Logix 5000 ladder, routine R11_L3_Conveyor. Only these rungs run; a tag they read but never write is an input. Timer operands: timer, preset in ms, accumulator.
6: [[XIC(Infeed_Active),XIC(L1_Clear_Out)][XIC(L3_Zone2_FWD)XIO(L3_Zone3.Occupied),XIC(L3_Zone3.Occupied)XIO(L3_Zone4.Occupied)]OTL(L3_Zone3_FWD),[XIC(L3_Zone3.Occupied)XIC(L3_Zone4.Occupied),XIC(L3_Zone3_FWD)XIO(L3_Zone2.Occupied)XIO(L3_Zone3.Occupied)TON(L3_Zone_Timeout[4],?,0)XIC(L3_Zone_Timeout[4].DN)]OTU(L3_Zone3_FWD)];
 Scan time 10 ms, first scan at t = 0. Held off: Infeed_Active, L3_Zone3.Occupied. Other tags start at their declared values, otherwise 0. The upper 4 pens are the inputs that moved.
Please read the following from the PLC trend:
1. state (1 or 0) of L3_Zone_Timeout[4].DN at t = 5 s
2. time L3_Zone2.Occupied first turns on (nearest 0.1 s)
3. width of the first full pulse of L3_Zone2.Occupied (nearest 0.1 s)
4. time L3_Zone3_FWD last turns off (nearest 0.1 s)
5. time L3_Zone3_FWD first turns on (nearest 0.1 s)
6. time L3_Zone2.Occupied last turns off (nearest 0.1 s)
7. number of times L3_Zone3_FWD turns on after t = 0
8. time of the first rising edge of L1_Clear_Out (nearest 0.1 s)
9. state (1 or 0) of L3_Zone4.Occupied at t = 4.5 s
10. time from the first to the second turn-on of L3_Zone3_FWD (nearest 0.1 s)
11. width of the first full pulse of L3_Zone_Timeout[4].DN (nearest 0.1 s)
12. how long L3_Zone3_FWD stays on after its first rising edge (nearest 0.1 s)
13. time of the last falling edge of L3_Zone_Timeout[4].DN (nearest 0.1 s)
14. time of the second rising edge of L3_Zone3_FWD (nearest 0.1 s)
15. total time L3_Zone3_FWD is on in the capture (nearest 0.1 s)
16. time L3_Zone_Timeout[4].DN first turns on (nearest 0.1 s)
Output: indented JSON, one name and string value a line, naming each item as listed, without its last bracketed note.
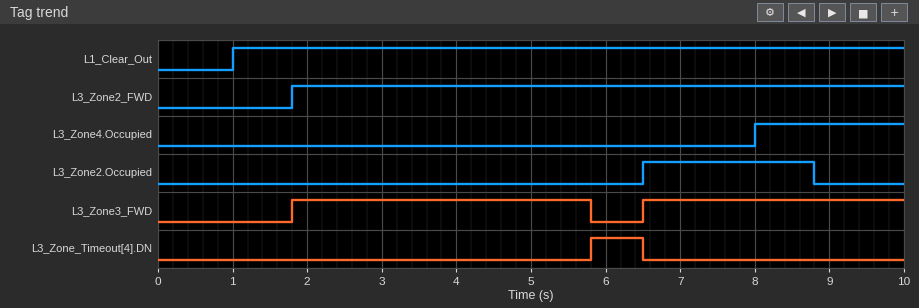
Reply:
{
  "state (1 or 0) of L3_Zone_Timeout[4].DN at t = 5 s": "0",
  "time L3_Zone2.Occupied first turns on": "6.5 s",
  "width of the first full pulse of L3_Zone2.Occupied": "2.3 s",
  "time L3_Zone3_FWD last turns off": "5.8 s",
  "time L3_Zone3_FWD first turns on": "1.8 s",
  "time L3_Zone2.Occupied last turns off": "8.8 s",
  "number of times L3_Zone3_FWD turns on after t = 0": "2",
  "time of the first rising edge of L1_Clear_Out": "1.0 s",
  "state (1 or 0) of L3_Zone4.Occupied at t = 4.5 s": "0",
  "time from the first to the second turn-on of L3_Zone3_FWD": "4.7 s",
  "width of the first full pulse of L3_Zone_Timeout[4].DN": "0.7 s",
  "how long L3_Zone3_FWD stays on after its first rising edge": "4.0 s",
  "time of the last falling edge of L3_Zone_Timeout[4].DN": "6.5 s",
  "time of the second rising edge of L3_Zone3_FWD": "6.5 s",
  "total time L3_Zone3_FWD is on in the capture": "7.5 s",
  "time L3_Zone_Timeout[4].DN first turns on": "5.8 s"
}
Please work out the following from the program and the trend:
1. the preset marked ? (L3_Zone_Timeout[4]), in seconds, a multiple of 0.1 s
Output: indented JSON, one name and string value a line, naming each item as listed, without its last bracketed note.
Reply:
{
  "the preset marked ? (L3_Zone_Timeout[4]), in seconds, a multiple of 0.1 s": "4.0 s"
}
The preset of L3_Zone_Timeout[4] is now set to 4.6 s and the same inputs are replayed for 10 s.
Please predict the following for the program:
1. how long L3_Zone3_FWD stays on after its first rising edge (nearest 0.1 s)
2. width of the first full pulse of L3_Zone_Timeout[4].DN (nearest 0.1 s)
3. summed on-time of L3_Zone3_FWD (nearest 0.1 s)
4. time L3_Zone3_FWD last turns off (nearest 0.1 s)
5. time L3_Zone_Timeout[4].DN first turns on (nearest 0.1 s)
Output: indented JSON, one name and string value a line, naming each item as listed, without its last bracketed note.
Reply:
{
  "how long L3_Zone3_FWD stays on after its first rising edge": "4.6 s",
  "width of the first full pulse of L3_Zone_Timeout[4].DN": "0.1 s",
  "summed on-time of L3_Zone3_FWD": "8.1 s",
  "time L3_Zone3_FWD last turns off": "6.4 s",
  "time L3_Zone_Timeout[4].DN first turns on": "6.4 s"
}
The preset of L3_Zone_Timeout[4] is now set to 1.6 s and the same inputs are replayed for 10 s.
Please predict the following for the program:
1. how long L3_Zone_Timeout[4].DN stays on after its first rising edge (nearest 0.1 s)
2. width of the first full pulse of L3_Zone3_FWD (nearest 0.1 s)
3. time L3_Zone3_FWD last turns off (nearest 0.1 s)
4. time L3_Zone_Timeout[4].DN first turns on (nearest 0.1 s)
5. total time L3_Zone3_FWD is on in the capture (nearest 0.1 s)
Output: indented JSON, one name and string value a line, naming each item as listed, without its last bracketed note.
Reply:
{
  "how long L3_Zone_Timeout[4].DN stays on after its first rising edge": "3.1 s",
  "width of the first full pulse of L3_Zone3_FWD": "1.6 s",
  "time L3_Zone3_FWD last turns off": "3.4 s",
  "time L3_Zone_Timeout[4].DN first turns on": "3.4 s",
  "total time L3_Zone3_FWD is on in the capture": "5.1 s"
}
